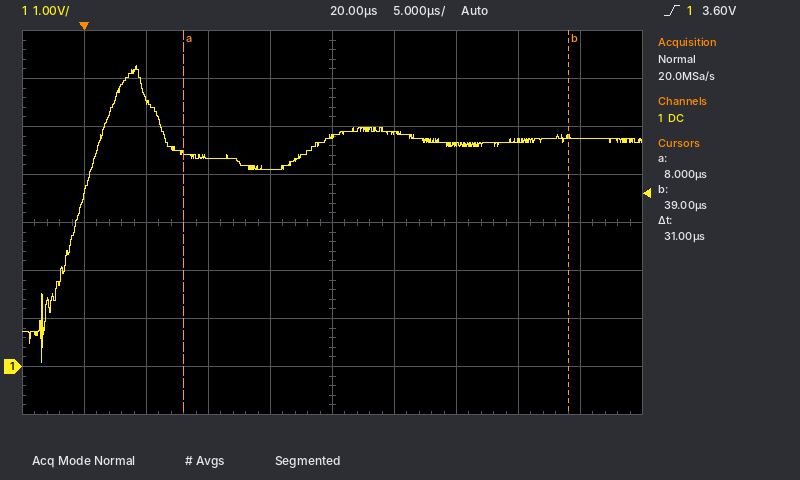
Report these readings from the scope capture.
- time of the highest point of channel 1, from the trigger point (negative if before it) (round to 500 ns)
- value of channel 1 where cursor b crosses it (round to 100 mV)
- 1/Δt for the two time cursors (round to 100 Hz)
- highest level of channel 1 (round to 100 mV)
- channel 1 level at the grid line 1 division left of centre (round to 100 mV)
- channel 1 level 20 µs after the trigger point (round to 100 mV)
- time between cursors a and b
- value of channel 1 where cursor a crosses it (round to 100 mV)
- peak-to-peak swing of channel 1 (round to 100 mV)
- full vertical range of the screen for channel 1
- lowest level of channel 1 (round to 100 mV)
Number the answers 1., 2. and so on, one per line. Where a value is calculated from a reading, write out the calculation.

1. +4.0 µs
2. 4.8 V
3. 1 / 31 µs ≈ 32.3 kHz
4. 6.3 V
5. 4.1 V
6. 4.8 V
7. 31 µs
8. 4.5 V
9. 6.3 V − (100 mV) = 6.2 V
10. 8 V
11. 100 mV
